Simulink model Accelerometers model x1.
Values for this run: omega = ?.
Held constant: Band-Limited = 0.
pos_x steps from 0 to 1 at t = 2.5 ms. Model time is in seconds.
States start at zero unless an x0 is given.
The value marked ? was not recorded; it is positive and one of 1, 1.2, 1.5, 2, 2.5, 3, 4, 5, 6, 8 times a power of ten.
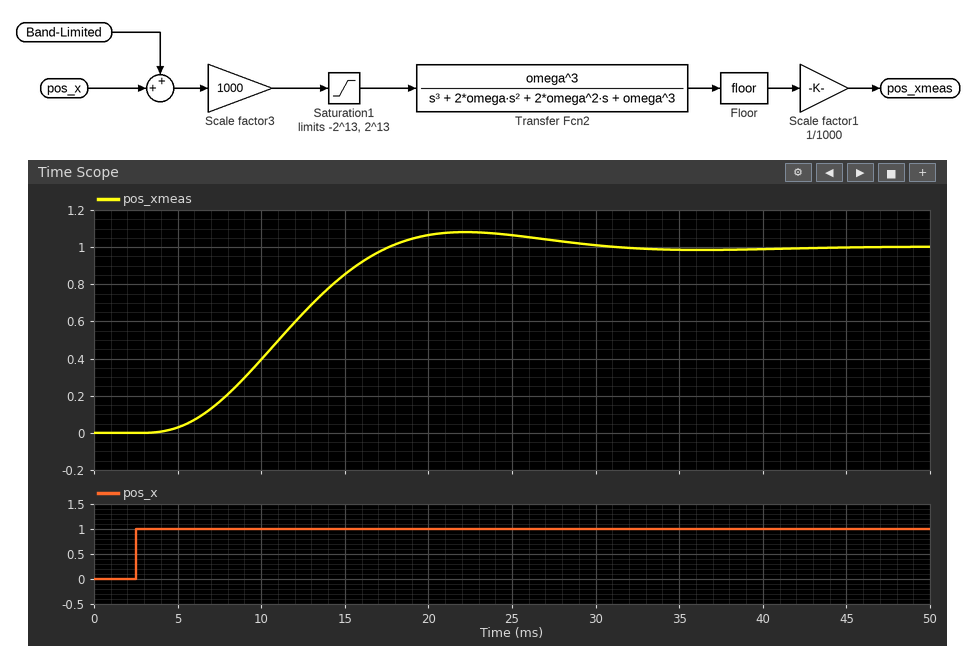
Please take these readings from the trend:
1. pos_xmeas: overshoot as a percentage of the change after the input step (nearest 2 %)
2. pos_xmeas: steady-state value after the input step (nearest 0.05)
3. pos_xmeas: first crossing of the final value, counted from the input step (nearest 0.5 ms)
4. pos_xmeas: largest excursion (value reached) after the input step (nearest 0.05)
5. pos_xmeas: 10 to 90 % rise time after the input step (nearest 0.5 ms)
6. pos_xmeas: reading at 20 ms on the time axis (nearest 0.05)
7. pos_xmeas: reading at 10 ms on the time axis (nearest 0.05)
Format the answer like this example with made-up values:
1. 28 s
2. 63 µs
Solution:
1. 8 %
2. 1.00
3. 15.0 ms
4. 1.10
5. 9.0 ms
6. 1.05
7. 0.40
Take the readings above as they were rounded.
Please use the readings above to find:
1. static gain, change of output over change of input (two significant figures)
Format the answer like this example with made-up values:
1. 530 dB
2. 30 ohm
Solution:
1. 1.0
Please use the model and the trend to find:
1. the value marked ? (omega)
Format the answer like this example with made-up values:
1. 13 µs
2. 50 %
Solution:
1. 250
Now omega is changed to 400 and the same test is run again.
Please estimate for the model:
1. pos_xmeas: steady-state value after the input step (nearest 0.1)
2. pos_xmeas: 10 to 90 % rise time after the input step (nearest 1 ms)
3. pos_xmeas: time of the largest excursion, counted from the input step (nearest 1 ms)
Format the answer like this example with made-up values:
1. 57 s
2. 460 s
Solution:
1. 1.0
2. 6 ms
3. 12 ms
